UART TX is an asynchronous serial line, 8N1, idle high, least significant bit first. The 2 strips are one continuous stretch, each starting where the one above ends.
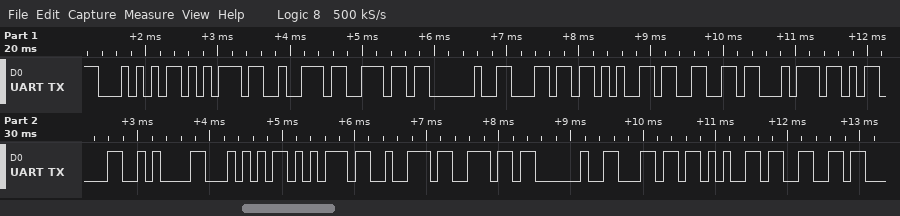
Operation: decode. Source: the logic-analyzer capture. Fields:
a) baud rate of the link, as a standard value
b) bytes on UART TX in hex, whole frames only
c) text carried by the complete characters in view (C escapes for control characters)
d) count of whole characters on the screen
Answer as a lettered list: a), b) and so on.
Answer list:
a) 9600 baud
b) 0x54 0x75 0x72 0x6E 0x20 0x6C 0x65 0x66 0x74 0x0D 0x0A 0x54 0x75 0x72 0x6E 0x20 0x6C 0x65 0x66
c) "Turn left\r\nTurn lef"
d) 19
